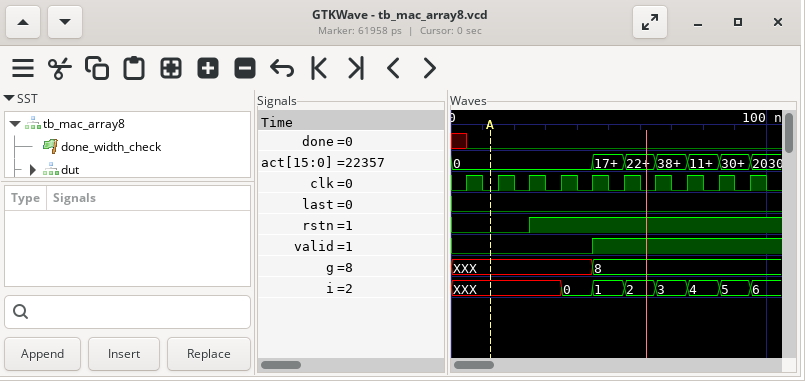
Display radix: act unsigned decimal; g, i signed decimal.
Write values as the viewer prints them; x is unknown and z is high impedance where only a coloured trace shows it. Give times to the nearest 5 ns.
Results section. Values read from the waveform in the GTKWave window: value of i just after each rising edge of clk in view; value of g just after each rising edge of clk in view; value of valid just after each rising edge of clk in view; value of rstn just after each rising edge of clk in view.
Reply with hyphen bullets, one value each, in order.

- XXX, XXX, XXX, 0, 1, 2, 3, 4, 5, 6
- XXX, XXX, XXX, XXX, 8, 8, 8, 8, 8, 8
- 0 0 0 0 1 1 1 1 1 1
- 0 0 1 1 1 1 1 1 1 1
